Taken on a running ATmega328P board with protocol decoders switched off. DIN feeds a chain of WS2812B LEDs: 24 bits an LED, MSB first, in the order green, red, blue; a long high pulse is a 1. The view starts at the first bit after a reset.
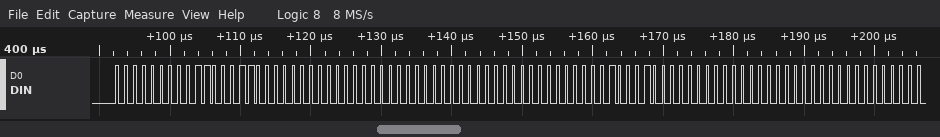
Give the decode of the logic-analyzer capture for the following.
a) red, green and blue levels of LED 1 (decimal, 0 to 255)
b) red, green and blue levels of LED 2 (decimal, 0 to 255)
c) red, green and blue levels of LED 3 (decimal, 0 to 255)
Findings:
99, 0, 0
0, 0, 0
136, 0, 0
